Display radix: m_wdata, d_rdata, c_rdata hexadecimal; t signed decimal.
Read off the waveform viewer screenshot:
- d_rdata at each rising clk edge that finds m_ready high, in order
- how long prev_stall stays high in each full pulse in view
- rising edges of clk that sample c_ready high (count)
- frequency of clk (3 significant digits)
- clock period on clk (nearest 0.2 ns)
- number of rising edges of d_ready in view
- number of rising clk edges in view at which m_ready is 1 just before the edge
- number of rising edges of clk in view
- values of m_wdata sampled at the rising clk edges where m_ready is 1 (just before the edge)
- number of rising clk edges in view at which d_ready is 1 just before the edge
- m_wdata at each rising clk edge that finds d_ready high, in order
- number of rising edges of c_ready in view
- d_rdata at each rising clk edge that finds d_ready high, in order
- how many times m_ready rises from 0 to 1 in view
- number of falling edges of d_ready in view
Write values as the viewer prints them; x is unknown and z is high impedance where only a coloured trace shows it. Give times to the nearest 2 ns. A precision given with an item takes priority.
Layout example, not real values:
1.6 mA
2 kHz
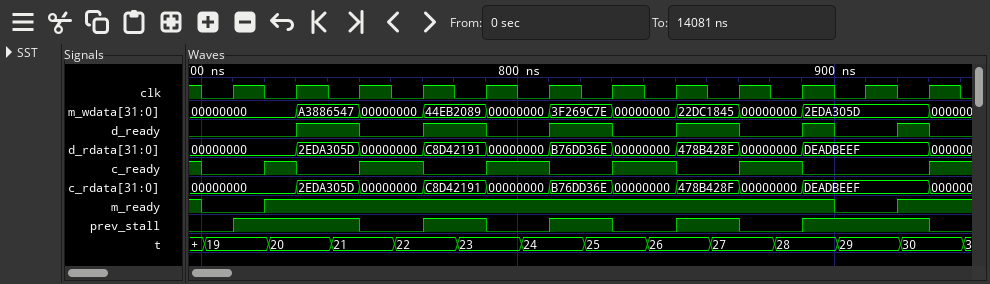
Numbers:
00000000, 2EDA305D, 00000000, C8D42191, 00000000, B76DD36E, 00000000, 478B428F, 00000000, DEADBEEF
40 ns, 20 ns, 20 ns, 20 ns, 40 ns
5
50.0 MHz
20 ns
6
10
12
00000000, A3886547, 00000000, 44EB2089, 00000000, 3F269C7E, 00000000, 22DC1845, 00000000, 2EDA305D
5
A3886547, 44EB2089, 3F269C7E, 22DC1845, 2EDA305D
6
2EDA305D, C8D42191, B76DD36E, 478B428F, DEADBEEF
2
6
